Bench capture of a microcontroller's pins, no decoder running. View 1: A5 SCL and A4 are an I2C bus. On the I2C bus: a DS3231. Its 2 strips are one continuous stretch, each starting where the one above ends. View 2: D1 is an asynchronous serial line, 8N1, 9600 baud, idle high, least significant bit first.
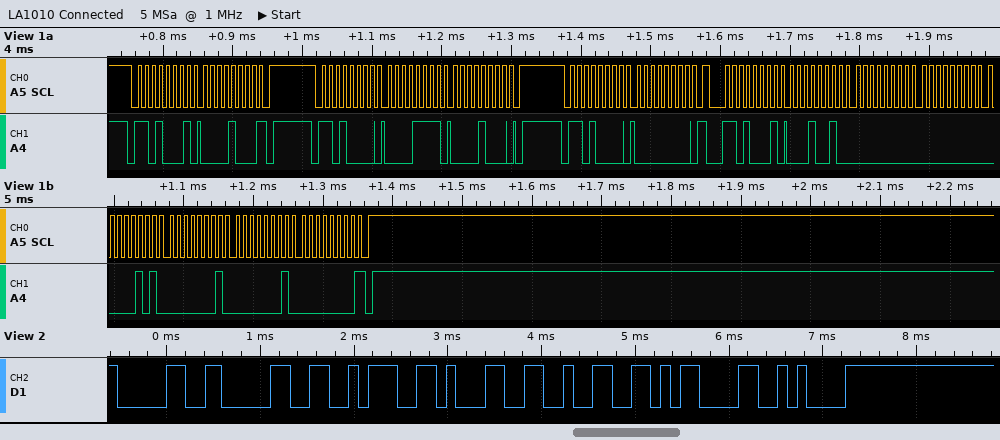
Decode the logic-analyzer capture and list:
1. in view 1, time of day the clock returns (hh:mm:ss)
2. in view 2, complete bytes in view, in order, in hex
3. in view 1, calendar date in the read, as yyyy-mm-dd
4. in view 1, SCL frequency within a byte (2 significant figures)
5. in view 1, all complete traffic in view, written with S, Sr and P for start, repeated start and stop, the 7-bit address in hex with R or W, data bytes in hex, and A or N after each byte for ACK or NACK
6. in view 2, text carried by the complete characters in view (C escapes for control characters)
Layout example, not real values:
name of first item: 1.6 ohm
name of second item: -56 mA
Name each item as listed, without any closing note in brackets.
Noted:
in view 1, time of day the clock returns: 00:00:12
in view 2, complete bytes in view, in order, in hex: 30 30 3A 31 32 0D 0A
in view 1, calendar date in the read, as yyyy-mm-dd: 2000-01-01
in view 1, SCL frequency within a byte: 100 kHz
in view 1, all complete traffic in view, written with S, Sr and P for start, repeated start and stop, the 7-bit address in hex with R or W, data bytes in hex, and A or N after each byte for ACK or NACK: S 68R A 08 N P S 68W A 0F A 08 A P S 68W A 00 A Sr 68R A 12 A 00 A 00 A 05 A 01 A 01 A 00 N P
in view 2, text carried by the complete characters in view: "00:12\r\n"
